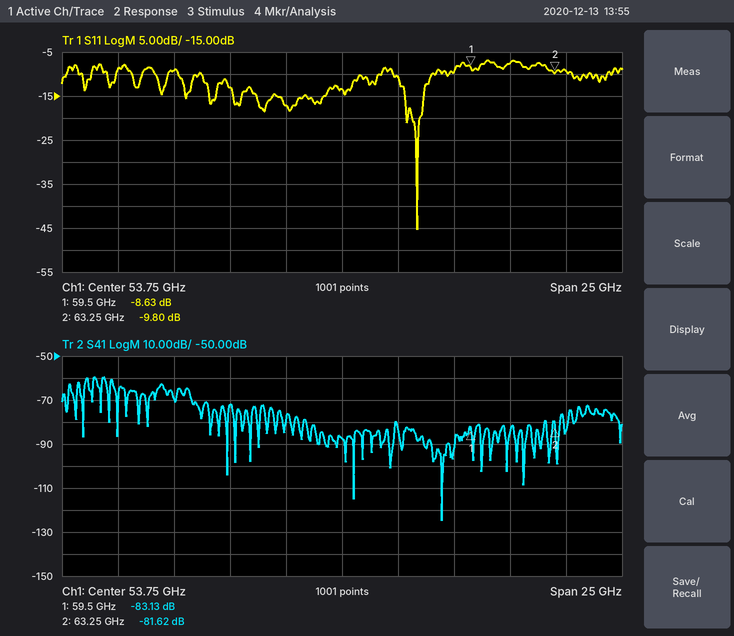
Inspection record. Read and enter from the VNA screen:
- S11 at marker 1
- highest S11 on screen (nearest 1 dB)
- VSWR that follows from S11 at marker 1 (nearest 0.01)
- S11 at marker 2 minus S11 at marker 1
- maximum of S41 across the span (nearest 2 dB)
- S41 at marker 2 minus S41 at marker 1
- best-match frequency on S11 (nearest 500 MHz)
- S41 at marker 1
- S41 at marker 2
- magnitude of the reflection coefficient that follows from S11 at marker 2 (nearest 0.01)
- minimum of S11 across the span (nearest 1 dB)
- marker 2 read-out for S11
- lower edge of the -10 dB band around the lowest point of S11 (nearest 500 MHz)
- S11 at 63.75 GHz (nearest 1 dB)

-8.63 dB
-7 dB
2.18
-1.17 dB
-60 dB
1.51 dB
57.0 GHz
-83.13 dB
-81.62 dB
0.32
-45 dB
-9.80 dB
56.0 GHz
-9 dB
